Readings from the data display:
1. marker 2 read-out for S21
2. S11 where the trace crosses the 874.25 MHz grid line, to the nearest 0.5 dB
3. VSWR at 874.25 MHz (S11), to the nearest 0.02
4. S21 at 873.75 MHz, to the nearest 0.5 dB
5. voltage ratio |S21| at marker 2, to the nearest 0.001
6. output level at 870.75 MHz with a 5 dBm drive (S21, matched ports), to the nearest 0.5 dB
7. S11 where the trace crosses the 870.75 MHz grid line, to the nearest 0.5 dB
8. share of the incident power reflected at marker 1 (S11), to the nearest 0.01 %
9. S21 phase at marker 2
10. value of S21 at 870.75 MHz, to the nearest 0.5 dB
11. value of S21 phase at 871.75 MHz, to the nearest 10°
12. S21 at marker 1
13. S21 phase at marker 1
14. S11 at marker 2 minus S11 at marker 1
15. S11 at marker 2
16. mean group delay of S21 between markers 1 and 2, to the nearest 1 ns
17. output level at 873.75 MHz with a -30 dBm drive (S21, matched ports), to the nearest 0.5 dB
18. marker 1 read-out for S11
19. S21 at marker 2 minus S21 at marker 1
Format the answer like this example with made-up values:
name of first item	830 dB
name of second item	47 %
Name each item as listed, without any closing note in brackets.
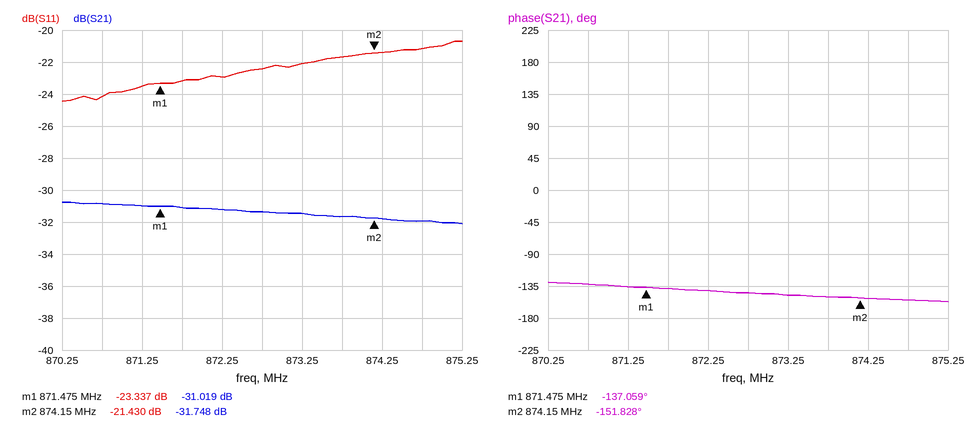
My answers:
marker 2 read-out for S21	-31.748 dB
S11 where the trace crosses the 874.25 MHz grid line, to the nearest 0.5 dB	-21.5 dB
VSWR at 874.25 MHz (S11), to the nearest 0.02	1.18
S21 at 873.75 MHz, to the nearest 0.5 dB	-31.5 dB
voltage ratio |S21| at marker 2, to the nearest 0.001	0.026
output level at 870.75 MHz with a 5 dBm drive (S21, matched ports), to the nearest 0.5 dB	-26.0 dBm
S11 where the trace crosses the 870.75 MHz grid line, to the nearest 0.5 dB	-24.0 dB
share of the incident power reflected at marker 1 (S11), to the nearest 0.01 %	0.46 %
S21 phase at marker 2	-151.828°
value of S21 at 870.75 MHz, to the nearest 0.5 dB	-31.0 dB
value of S21 phase at 871.75 MHz, to the nearest 10°	-140°
S21 at marker 1	-31.019 dB
S21 phase at marker 1	-137.059°
S11 at marker 2 minus S11 at marker 1	1.907 dB
S11 at marker 2	-21.430 dB
mean group delay of S21 between markers 1 and 2, to the nearest 1 ns	15 ns
output level at 873.75 MHz with a -30 dBm drive (S21, matched ports), to the nearest 0.5 dB	-61.5 dBm
marker 1 read-out for S11	-23.337 dB
S21 at marker 2 minus S21 at marker 1	-0.729 dB
